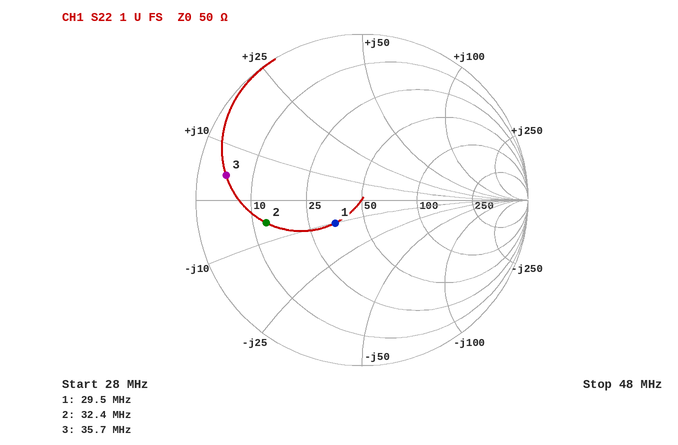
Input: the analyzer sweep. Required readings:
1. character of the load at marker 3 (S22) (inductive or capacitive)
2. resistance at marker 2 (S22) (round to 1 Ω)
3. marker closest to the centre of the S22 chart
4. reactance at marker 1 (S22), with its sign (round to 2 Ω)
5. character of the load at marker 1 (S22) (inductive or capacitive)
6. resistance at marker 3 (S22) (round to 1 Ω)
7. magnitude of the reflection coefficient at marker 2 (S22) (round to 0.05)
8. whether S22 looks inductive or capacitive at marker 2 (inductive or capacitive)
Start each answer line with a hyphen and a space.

- inductive
- 13 Ω
- marker 1
- -10 Ω
- capacitive
- 5 Ω
- 0.60
- capacitive
